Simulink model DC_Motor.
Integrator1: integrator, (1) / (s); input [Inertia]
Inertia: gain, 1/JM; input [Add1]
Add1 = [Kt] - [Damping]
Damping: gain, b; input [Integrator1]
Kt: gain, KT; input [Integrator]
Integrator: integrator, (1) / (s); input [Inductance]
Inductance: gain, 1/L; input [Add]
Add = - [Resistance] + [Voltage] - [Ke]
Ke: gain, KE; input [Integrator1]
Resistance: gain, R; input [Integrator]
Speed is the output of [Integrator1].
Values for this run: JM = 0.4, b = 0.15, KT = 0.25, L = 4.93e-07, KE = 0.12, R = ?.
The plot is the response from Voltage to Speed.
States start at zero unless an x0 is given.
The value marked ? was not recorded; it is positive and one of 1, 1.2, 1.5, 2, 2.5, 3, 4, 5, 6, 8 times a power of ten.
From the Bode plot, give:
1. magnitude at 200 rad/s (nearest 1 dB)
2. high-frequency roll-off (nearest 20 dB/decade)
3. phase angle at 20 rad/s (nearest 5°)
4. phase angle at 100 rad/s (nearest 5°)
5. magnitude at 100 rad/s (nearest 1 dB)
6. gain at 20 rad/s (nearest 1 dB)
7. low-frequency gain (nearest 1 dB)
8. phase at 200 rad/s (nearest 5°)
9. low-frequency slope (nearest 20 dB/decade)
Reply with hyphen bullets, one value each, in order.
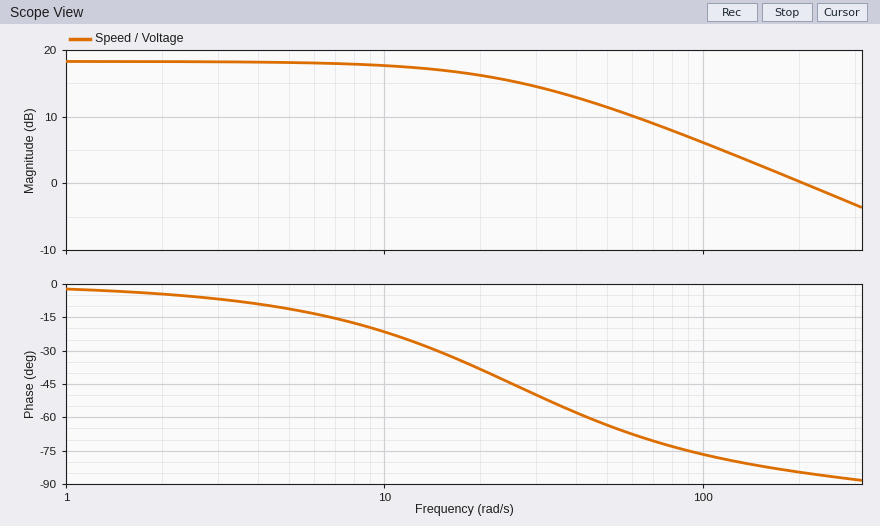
- 0 dB
- -20 dB/decade
- -40°
- -75°
- 6 dB
- 16 dB
- 18 dB
- -85°
- 0 dB/decade
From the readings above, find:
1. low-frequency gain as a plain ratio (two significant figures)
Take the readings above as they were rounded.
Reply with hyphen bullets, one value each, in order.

- 7.9
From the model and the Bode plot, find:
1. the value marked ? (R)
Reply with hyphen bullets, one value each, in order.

- 0.003
